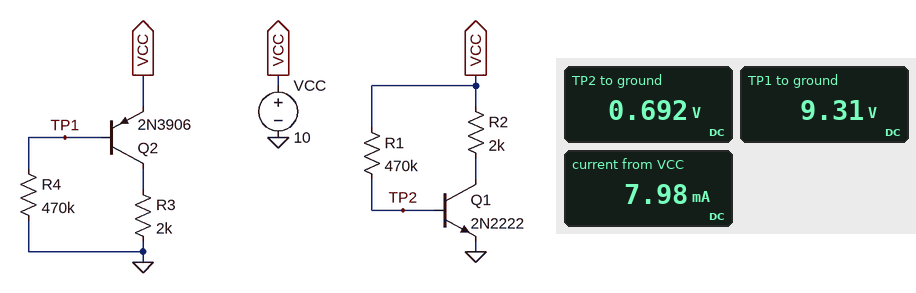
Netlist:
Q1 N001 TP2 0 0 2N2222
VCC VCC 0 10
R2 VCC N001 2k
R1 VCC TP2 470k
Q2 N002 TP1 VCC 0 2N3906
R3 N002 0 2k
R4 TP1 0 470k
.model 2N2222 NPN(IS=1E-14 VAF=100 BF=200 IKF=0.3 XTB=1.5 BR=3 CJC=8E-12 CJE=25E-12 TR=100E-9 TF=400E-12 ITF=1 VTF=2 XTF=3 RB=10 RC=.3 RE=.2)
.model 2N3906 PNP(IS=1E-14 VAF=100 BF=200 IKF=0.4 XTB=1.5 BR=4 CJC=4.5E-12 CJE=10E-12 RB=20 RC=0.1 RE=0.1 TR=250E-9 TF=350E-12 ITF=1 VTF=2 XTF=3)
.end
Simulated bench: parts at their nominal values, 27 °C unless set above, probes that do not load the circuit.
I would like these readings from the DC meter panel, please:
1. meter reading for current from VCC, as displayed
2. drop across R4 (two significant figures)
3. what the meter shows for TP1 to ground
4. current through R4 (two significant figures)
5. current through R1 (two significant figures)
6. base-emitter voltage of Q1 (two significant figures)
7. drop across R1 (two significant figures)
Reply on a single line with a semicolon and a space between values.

7.98 mA; 9.3 V; 9.31 V; 20 µA; 20 µA; 690 mV; 9.3 V
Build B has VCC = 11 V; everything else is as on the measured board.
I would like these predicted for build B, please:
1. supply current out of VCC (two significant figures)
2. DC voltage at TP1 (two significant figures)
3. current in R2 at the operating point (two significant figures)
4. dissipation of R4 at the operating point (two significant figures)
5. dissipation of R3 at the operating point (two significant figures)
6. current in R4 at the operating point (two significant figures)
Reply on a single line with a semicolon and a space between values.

8.8 mA; 10 V; 4.4 mA; 230 µW; 39 mW; 22 µA
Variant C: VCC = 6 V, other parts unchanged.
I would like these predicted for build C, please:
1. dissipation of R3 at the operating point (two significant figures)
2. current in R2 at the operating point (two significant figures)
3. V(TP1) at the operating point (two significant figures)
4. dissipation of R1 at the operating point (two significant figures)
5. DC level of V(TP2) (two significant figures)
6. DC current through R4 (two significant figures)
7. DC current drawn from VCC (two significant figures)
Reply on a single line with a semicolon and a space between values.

10 mW; 2.3 mA; 5.3 V; 60 µW; 680 mV; 11 µA; 4.6 mA
